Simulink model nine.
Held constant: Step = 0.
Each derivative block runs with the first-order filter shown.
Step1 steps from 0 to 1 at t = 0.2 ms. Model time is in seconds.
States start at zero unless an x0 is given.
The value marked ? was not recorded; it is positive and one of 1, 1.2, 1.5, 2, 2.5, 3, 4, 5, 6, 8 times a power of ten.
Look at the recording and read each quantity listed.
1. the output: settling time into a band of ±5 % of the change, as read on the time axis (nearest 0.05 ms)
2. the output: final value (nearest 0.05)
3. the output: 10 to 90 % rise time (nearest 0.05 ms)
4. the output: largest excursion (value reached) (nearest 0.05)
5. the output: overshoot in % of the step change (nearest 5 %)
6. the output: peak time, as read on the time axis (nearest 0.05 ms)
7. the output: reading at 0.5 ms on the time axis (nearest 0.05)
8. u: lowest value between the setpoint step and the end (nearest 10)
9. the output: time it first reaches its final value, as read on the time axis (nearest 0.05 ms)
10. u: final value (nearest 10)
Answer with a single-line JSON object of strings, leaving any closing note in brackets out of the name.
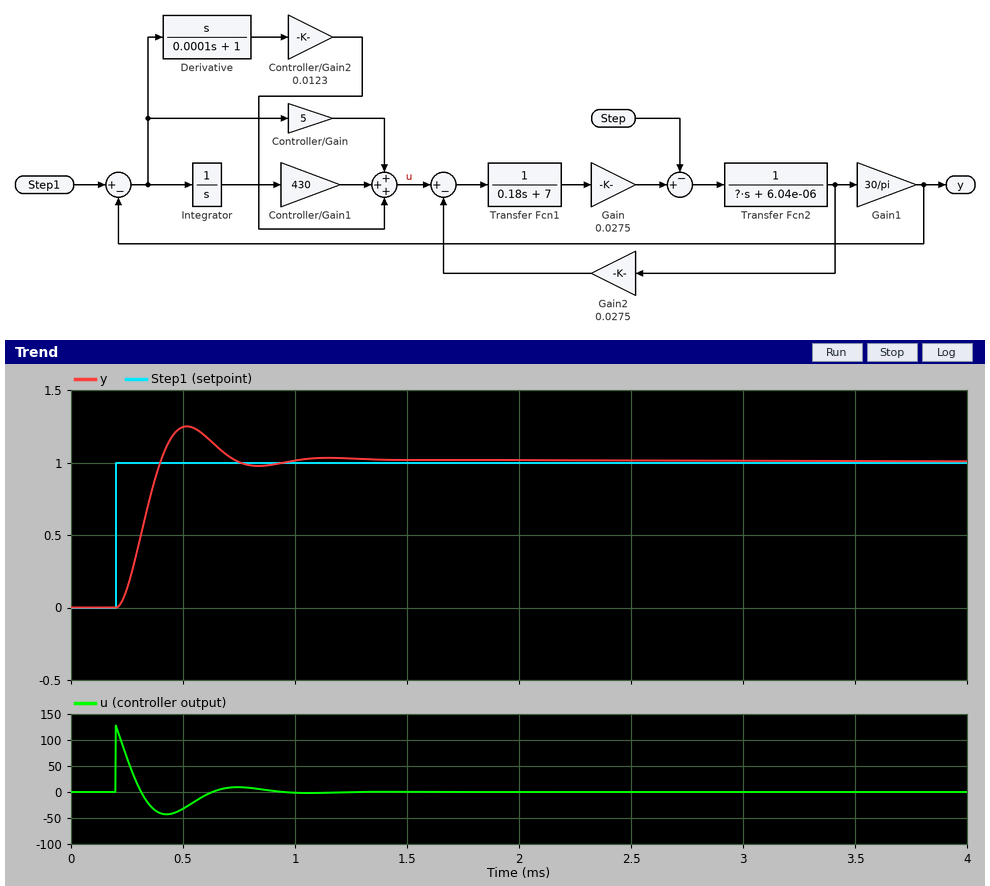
{"the output: settling time into a band of ±5 % of the change, as read on the time axis": "0.70 ms", "the output: final value": "1.00", "the output: 10 to 90 % rise time": "0.15 ms", "the output: largest excursion (value reached)": "1.25", "the output: overshoot in % of the step change": "25 %", "the output: peak time, as read on the time axis": "0.50 ms", "the output: reading at 0.5 ms on the time axis": "1.25", "u: lowest value between the setpoint step and the end": "-40", "the output: time it first reaches its final value, as read on the time axis": "0.40 ms", "u: final value": "0"}
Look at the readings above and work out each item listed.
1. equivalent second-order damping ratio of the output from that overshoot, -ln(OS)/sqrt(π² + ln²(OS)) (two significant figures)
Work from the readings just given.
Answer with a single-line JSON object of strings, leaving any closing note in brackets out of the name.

{"equivalent second-order damping ratio of the output from that overshoot, -ln(OS)/sqrt(π² + ln²(OS))": "0.40"}
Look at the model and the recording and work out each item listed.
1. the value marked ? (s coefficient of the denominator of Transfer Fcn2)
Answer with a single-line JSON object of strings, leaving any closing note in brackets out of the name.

{"the value marked ?": "1.5e-06"}
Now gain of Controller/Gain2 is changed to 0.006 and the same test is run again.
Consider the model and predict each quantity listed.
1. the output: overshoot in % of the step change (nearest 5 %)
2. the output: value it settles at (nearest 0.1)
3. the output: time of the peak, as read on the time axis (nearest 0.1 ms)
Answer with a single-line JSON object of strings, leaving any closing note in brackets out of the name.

{"the output: overshoot in % of the step change": "20 %", "the output: value it settles at": "1.0", "the output: time of the peak, as read on the time axis": "0.7 ms"}
